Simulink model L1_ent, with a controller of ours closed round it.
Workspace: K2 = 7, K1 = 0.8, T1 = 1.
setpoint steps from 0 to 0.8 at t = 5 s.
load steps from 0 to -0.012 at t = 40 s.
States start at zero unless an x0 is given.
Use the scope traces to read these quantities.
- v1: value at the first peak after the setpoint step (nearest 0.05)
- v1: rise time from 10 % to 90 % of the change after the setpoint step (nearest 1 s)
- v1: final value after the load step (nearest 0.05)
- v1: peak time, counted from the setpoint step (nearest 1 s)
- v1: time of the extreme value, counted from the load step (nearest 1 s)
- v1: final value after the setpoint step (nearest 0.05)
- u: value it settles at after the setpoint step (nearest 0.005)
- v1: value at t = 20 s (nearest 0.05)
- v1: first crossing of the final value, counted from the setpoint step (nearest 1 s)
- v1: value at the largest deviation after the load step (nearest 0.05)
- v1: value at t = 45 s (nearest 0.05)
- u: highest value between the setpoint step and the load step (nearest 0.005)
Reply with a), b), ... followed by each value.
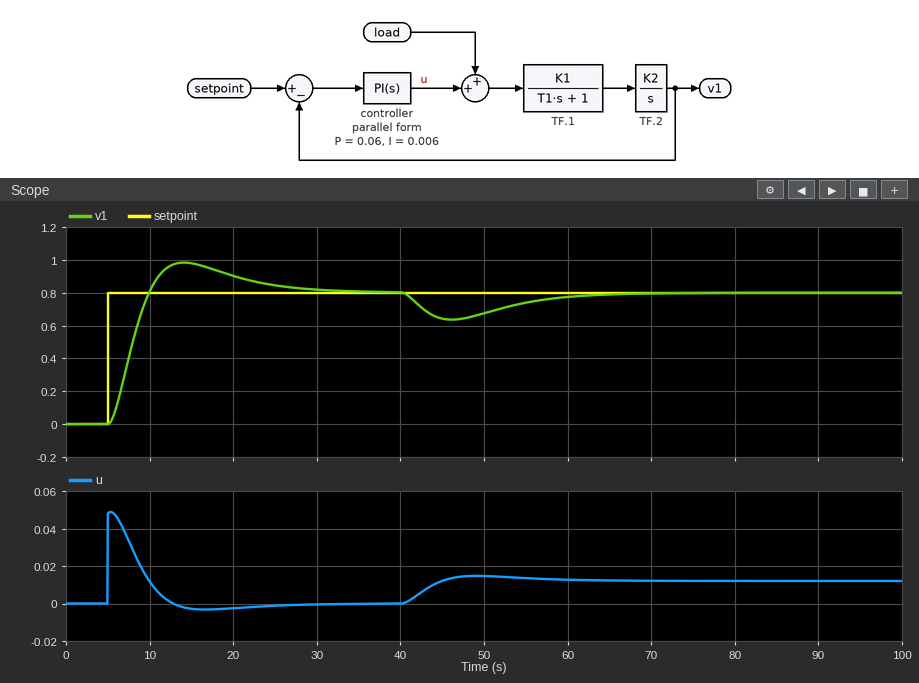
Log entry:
a) 1.00
b) 3 s
c) 0.80
d) 9 s
e) 6 s
f) 0.80
g) 0.000
h) 0.90
i) 5 s
j) 0.65
k) 0.65
l) 0.050
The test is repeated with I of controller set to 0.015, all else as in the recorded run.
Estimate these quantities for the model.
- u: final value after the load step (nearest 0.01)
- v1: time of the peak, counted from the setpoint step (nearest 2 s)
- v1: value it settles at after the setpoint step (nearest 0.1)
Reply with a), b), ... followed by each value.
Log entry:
a) 0.01
b) 8 s
c) 0.8
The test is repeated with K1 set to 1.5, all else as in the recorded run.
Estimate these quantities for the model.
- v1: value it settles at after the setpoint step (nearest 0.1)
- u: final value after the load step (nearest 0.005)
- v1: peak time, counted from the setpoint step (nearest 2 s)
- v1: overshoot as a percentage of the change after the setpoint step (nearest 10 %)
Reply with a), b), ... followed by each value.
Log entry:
a) 0.8
b) 0.010
c) 6 s
d) 20 %
